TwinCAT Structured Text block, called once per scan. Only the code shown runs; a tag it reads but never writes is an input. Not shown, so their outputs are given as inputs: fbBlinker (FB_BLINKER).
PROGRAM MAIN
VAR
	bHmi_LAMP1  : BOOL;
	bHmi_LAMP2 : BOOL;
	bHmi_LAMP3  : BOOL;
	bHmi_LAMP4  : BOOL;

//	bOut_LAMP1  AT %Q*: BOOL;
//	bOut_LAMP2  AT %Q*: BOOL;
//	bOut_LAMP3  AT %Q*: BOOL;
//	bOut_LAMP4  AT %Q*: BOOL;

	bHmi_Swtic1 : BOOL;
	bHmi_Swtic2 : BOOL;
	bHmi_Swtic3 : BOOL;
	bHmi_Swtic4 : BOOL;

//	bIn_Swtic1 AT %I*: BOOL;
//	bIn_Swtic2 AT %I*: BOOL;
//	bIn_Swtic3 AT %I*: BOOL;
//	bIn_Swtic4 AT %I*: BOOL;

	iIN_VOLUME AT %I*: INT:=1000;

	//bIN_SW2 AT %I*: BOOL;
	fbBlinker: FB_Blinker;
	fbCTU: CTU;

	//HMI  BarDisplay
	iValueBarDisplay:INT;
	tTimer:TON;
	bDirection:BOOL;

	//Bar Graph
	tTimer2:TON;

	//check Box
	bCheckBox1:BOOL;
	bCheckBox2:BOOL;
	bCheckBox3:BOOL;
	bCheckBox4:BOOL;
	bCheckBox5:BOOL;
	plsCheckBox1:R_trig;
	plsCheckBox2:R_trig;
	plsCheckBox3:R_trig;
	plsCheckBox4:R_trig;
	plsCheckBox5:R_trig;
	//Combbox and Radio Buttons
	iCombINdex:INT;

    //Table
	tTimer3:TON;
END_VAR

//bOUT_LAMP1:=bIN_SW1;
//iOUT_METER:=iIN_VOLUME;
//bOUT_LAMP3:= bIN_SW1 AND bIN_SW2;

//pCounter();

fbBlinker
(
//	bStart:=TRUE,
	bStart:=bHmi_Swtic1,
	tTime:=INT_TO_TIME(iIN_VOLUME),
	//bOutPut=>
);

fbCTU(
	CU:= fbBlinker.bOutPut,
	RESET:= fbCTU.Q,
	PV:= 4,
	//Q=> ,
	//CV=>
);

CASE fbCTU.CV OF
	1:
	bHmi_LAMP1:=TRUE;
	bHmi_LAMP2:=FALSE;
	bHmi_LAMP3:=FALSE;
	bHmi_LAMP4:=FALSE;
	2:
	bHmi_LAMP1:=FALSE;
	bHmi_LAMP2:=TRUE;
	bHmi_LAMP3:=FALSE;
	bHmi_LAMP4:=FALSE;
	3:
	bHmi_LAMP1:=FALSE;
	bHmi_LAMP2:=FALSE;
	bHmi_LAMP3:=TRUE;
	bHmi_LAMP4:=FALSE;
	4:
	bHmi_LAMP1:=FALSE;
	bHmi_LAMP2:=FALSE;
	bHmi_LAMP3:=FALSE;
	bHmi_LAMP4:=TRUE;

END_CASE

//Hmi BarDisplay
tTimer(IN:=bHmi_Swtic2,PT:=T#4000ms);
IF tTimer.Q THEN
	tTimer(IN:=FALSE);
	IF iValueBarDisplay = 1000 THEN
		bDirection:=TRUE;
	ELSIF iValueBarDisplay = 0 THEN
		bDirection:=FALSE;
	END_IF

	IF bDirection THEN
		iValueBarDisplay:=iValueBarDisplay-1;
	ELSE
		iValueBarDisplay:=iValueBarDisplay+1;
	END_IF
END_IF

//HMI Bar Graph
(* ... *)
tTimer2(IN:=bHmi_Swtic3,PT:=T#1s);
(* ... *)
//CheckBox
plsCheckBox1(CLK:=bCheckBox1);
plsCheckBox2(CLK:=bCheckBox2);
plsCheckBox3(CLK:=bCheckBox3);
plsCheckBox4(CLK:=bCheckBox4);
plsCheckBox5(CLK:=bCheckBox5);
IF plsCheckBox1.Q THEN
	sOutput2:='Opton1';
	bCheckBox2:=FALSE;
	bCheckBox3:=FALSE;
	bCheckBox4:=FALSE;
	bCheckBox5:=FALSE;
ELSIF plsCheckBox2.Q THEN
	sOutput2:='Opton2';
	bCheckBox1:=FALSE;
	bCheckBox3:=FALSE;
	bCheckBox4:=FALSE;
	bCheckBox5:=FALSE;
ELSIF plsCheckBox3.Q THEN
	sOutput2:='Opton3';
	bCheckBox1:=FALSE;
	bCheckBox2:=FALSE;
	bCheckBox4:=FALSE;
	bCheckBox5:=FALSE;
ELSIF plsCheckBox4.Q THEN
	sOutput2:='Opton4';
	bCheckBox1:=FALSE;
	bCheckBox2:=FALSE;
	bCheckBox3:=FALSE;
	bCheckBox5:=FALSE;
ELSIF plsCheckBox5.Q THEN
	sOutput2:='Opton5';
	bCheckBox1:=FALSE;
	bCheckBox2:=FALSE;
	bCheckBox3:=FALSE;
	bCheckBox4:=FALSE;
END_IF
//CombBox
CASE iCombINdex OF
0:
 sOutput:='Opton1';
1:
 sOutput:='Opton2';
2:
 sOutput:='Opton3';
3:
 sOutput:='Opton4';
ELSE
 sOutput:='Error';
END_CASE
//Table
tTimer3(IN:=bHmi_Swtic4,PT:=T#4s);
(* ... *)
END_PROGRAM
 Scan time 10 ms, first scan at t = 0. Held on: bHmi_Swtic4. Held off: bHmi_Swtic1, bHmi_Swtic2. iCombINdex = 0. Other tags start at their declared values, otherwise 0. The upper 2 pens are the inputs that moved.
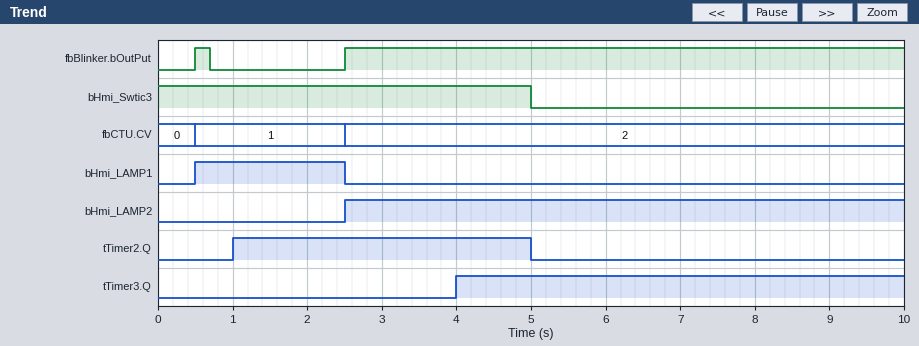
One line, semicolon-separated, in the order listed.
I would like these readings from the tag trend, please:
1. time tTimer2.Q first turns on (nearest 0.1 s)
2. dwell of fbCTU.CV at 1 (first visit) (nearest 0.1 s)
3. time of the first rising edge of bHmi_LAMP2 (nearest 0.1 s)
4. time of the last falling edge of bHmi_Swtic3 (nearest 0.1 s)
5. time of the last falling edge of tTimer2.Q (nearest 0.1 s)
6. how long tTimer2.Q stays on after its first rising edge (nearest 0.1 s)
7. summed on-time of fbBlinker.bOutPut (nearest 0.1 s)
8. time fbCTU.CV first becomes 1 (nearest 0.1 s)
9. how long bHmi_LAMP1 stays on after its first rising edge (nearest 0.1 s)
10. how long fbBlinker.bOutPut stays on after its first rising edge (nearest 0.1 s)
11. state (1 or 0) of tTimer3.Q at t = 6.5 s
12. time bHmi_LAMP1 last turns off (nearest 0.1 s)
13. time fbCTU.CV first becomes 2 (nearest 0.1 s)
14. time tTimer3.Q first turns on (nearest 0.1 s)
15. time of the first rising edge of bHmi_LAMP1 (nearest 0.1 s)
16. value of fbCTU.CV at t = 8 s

1.0 s; 2.0 s; 2.5 s; 5.0 s; 5.0 s; 4.0 s; 7.7 s; 0.5 s; 2.0 s; 0.2 s; 1; 2.5 s; 2.5 s; 4.0 s; 0.5 s; 2
